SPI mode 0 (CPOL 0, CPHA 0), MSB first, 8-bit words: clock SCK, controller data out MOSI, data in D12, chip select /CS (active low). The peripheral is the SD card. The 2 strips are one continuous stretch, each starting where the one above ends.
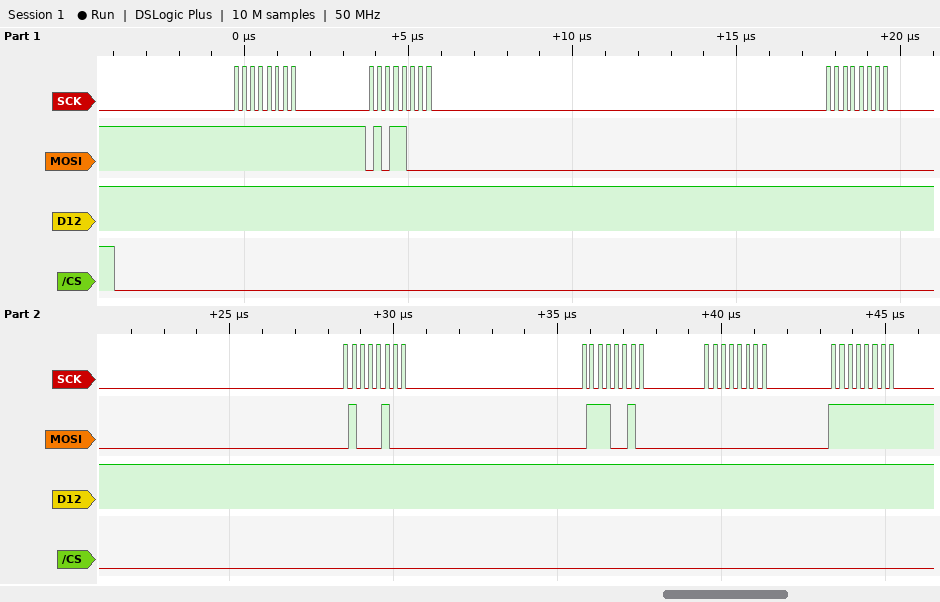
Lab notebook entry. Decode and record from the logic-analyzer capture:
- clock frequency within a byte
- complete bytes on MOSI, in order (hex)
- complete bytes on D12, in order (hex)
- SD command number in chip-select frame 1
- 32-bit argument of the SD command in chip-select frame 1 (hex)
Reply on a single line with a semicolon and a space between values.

4 MHz; FF 58 00 44 72 00 FF; FF FF FF FF FF FF FF; CMD24; 0x00447200
